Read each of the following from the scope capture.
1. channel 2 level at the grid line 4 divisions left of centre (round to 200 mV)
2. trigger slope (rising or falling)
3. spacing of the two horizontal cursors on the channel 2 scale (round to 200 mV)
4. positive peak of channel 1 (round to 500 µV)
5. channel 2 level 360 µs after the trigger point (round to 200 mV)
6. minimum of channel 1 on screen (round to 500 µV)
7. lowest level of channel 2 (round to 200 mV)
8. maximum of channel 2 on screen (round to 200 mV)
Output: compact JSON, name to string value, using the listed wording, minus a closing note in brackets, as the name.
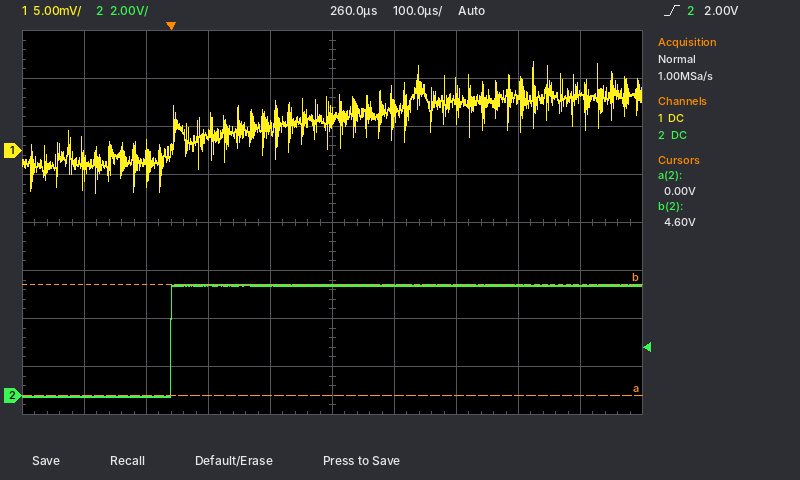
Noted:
{"channel 2 level at the grid line 4 divisions left of centre": "0.0 V", "trigger slope": "rising", "spacing of the two horizontal cursors on the channel 2 scale": "4.6 V", "positive peak of channel 1": "9.5 mV", "channel 2 level 360 µs after the trigger point": "4.6 V", "minimum of channel 1 on screen": "-4.5 mV", "lowest level of channel 2": "0.0 V", "maximum of channel 2 on screen": "4.6 V"}
